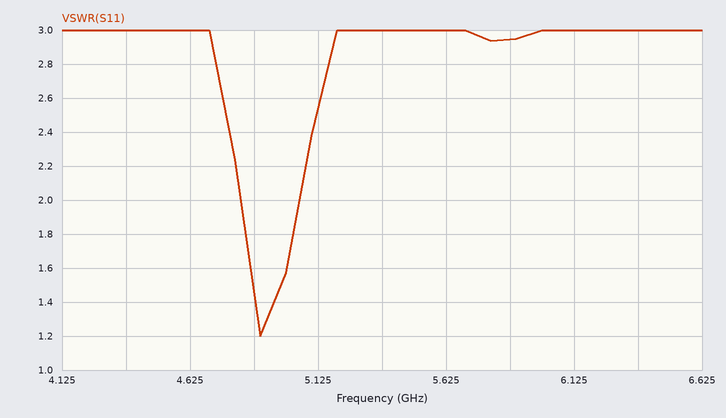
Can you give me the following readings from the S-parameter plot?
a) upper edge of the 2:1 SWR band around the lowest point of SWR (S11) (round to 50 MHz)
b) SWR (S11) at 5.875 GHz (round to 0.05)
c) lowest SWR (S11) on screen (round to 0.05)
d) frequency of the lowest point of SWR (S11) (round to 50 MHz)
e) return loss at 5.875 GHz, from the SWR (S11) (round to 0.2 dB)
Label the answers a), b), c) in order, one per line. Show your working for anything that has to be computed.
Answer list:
a) 5.05 GHz
b) 2.95
c) 1.20
d) 4.90 GHz
e) −20 log10((2.95 − 1)/(2.95 + 1)) ≈ 6.13 dB, so 6.2 dB to the nearest 0.2 dB
